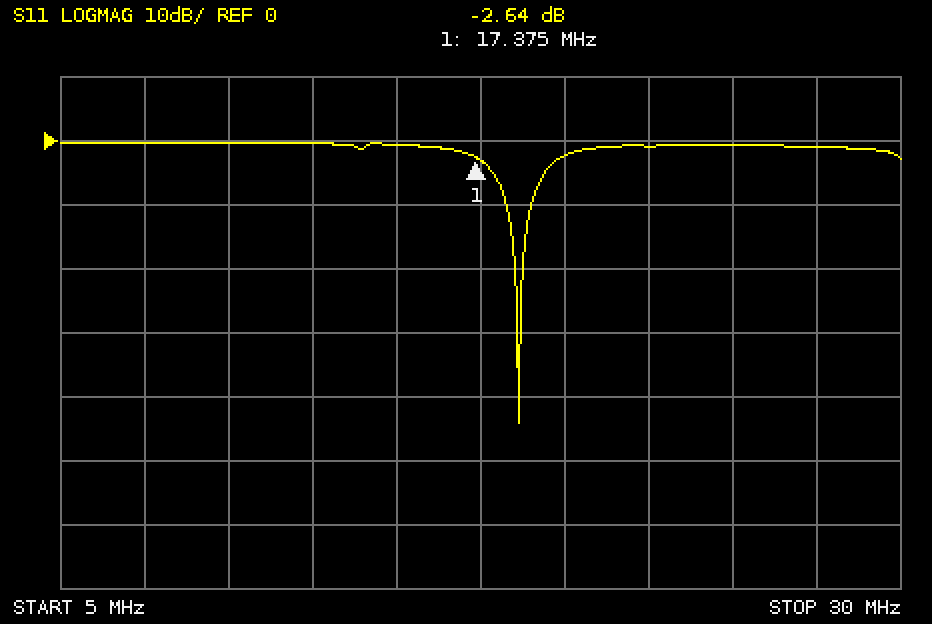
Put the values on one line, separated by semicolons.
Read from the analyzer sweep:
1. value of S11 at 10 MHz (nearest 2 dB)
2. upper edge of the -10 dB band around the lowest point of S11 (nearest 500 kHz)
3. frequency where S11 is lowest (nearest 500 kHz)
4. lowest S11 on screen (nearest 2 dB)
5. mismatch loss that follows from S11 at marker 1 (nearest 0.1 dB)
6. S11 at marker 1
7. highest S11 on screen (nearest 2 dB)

0 dB; 19.0 MHz; 18.5 MHz; -44 dB; 3.4 dB; -2.64 dB; 0 dB
